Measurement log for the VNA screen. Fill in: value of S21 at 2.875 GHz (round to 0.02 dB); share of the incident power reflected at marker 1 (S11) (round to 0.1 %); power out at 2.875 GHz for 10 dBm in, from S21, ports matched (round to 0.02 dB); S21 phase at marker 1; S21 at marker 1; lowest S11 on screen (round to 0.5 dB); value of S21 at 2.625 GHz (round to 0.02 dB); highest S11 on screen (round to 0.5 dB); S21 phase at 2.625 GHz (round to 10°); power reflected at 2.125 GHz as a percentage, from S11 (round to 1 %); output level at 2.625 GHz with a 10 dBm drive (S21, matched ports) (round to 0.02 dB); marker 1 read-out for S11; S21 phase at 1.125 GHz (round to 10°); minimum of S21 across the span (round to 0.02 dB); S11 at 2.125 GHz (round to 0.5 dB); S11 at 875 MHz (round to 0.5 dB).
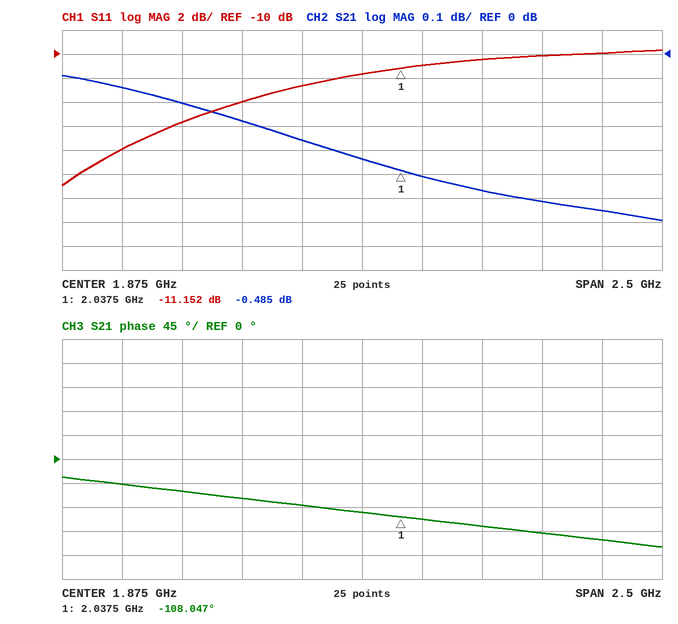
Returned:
-0.66 dB
7.7 %
9.34 dBm
-108.047°
-0.485 dB
-21.0 dB
-0.62 dB
-9.5 dB
-140°
8 %
9.38 dBm
-11.152 dB
-60°
-0.70 dB
-11.0 dB
-18.0 dB
